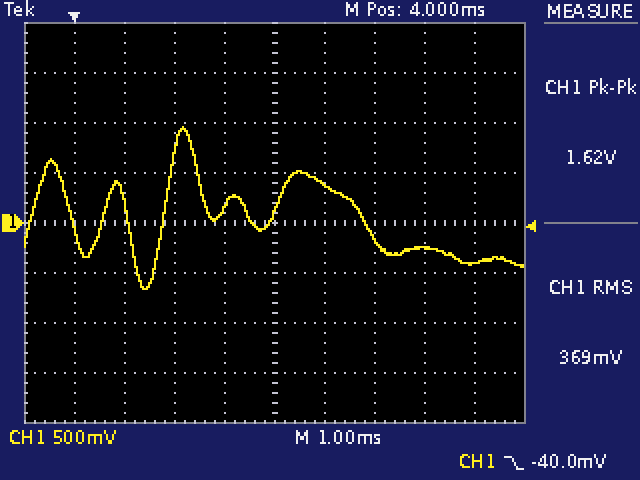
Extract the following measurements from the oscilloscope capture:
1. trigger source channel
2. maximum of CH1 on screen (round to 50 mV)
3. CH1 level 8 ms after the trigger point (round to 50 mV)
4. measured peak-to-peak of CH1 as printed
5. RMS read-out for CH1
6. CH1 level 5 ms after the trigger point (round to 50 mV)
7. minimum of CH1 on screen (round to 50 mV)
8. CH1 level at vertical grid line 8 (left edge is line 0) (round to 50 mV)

CH1
950 mV
-400 mV
1.62 V
369 mV
400 mV
-650 mV
-250 mV
